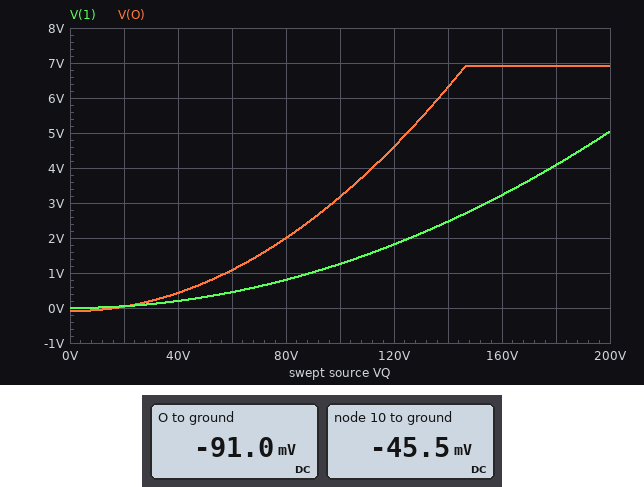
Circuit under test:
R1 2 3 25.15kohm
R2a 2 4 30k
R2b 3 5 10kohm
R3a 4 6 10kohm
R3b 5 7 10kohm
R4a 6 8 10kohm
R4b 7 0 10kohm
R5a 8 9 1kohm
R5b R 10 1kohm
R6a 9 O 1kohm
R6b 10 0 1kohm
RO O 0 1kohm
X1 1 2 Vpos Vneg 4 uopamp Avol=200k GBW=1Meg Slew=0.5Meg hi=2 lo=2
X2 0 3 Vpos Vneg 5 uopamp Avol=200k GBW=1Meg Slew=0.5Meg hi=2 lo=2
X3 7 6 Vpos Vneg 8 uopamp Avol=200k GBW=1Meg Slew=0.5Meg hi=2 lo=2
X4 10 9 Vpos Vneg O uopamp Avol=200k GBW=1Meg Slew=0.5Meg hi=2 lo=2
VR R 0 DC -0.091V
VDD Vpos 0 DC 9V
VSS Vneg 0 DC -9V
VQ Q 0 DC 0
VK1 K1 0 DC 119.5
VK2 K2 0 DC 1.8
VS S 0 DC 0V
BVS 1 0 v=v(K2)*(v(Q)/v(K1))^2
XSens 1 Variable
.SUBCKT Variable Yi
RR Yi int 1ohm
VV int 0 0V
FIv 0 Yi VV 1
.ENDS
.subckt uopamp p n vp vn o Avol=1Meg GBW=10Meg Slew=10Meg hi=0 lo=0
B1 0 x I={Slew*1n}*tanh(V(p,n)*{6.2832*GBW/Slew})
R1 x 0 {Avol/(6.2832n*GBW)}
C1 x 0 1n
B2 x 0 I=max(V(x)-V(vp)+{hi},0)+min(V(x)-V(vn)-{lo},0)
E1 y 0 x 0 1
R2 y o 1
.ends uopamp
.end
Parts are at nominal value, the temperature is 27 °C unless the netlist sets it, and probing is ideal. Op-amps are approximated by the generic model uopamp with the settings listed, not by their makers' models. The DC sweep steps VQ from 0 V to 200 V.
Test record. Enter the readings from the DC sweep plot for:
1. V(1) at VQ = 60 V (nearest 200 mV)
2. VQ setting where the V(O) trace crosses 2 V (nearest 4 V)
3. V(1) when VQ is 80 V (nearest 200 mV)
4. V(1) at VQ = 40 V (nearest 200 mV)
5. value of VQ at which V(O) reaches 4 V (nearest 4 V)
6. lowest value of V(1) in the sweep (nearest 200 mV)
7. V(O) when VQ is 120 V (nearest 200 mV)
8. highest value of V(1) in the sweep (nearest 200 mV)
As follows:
400 mV
80 V
800 mV
200 mV
112 V
0 V
4.6 V
5.0 V
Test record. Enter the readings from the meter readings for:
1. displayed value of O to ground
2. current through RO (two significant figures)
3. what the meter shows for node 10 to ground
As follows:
-91.0 mV
91 µA
-45.5 mV
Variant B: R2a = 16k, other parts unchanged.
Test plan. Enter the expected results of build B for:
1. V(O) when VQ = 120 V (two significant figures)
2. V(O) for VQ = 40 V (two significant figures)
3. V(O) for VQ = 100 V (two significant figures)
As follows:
3.6 V
320 mV
2.5 V
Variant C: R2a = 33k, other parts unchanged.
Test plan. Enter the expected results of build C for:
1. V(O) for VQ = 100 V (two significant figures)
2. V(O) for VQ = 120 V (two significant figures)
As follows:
3.3 V
4.8 V
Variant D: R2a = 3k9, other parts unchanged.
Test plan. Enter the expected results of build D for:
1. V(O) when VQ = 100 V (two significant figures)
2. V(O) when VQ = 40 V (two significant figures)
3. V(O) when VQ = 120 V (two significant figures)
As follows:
1.9 V
220 mV
2.7 V
